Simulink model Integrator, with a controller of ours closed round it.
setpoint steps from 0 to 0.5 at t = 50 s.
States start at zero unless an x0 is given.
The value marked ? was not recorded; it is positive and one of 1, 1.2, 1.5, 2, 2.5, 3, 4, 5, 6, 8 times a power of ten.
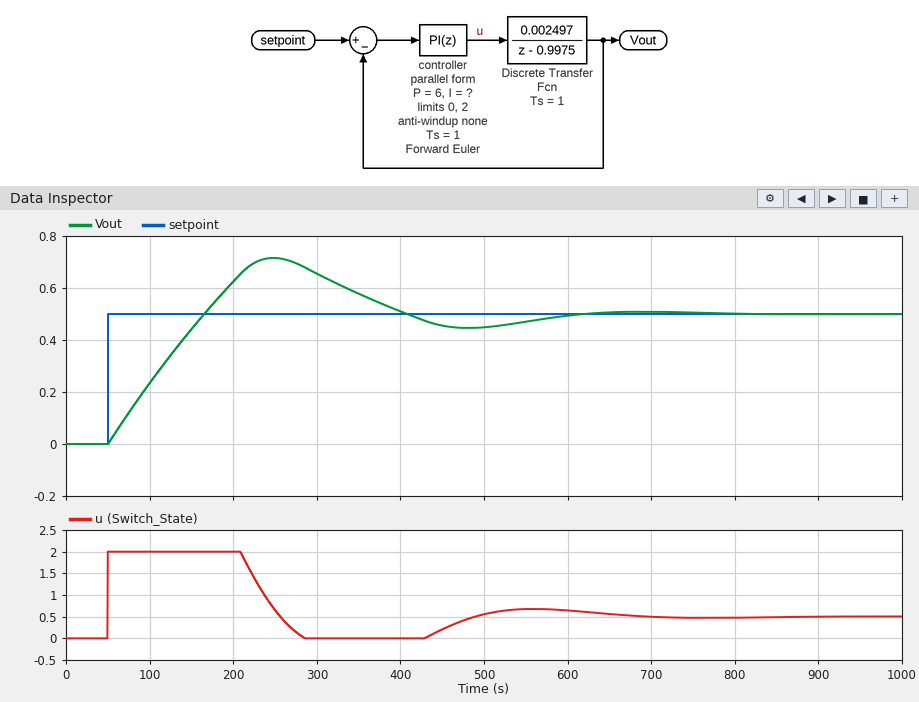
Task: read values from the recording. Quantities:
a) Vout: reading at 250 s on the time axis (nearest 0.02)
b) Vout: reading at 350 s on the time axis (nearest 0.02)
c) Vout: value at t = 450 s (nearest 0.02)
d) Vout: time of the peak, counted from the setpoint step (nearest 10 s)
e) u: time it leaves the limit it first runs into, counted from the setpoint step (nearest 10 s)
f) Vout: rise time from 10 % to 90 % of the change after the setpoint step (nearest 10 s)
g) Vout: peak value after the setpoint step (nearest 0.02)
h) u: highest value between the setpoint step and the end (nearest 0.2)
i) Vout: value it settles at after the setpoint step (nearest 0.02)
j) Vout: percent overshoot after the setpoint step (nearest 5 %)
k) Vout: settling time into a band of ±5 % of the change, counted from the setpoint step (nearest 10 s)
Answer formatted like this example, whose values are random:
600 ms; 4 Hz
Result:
0.72; 0.58; 0.46; 200 s; 160 s; 90 s; 0.72; 2.0; 0.50; 45 %; 510 s
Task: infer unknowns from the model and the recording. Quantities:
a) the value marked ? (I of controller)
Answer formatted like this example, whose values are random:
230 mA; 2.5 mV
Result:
0.12
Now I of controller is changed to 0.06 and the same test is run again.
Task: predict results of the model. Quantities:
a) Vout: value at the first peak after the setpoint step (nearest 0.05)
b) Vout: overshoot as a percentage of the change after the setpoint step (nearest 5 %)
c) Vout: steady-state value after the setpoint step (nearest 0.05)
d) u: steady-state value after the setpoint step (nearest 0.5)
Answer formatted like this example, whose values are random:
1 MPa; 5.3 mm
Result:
0.60; 20 %; 0.50; 0.5
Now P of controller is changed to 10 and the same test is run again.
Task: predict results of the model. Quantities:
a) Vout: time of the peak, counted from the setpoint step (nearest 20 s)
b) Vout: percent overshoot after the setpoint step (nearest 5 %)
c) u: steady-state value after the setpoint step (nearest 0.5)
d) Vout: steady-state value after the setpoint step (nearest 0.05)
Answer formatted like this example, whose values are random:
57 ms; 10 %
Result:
180 s; 35 %; 0.5; 0.50
